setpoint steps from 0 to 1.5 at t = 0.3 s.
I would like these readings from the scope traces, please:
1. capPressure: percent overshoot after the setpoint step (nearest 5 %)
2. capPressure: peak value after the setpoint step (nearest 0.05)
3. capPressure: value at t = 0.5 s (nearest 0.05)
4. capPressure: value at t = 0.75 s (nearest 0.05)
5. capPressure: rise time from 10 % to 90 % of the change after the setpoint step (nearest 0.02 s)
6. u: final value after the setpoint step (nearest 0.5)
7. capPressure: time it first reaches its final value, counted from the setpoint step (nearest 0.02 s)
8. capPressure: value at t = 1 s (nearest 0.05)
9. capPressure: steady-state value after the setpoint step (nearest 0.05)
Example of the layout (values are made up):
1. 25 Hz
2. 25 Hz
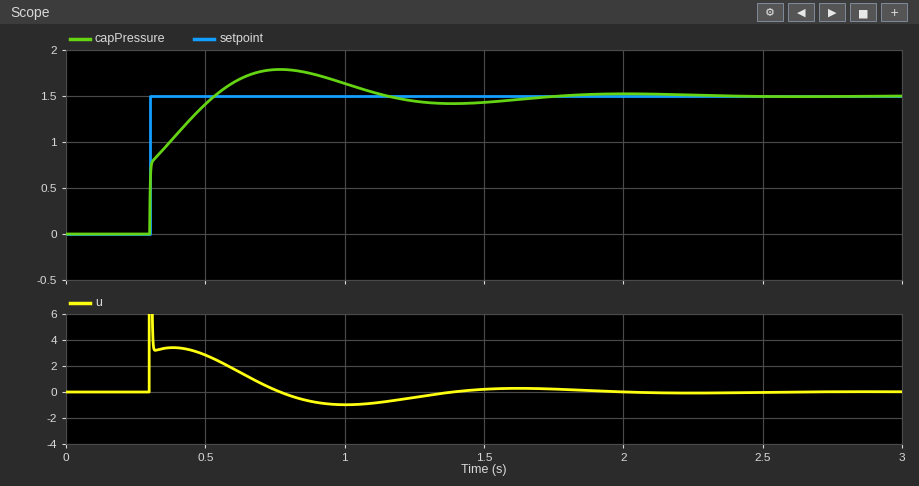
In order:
1. 20 %
2. 1.80
3. 1.40
4. 1.80
5. 0.18 s
6. 0.0
7. 0.24 s
8. 1.65
9. 1.50
